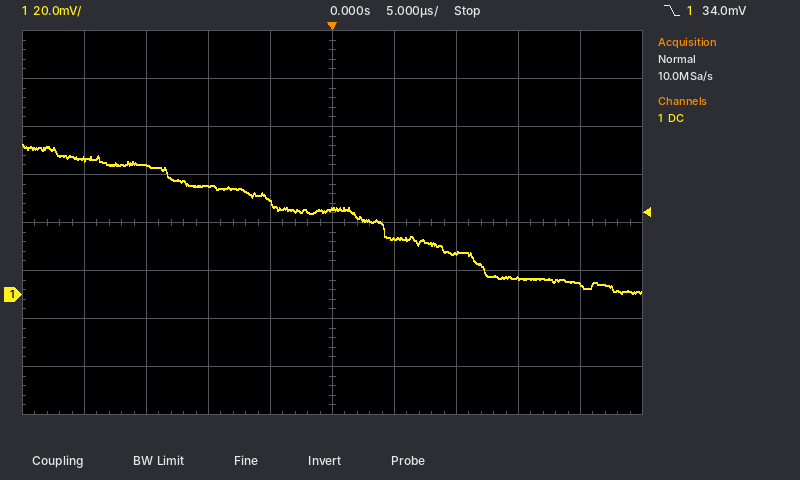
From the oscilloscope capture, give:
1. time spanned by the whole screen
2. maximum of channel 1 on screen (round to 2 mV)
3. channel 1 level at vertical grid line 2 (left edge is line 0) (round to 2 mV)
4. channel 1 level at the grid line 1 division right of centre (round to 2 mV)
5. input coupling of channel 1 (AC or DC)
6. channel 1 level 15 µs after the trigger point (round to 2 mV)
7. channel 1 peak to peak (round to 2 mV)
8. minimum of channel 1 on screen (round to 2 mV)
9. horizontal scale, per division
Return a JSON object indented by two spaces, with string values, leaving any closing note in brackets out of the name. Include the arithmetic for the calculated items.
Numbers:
{
  "time spanned by the whole screen": "50 µs",
  "maximum of channel 1 on screen": "62 mV",
  "channel 1 level at vertical grid line 2 (left edge is line 0)": "54 mV",
  "channel 1 level at the grid line 1 division right of centre": "24 mV",
  "input coupling of channel 1": "DC",
  "channel 1 level 15 µs after the trigger point": "6 mV",
  "channel 1 peak to peak": "62 mV − (0 mV) = 62 mV",
  "minimum of channel 1 on screen": "0 mV",
  "horizontal scale, per division": "5 µs"
}
